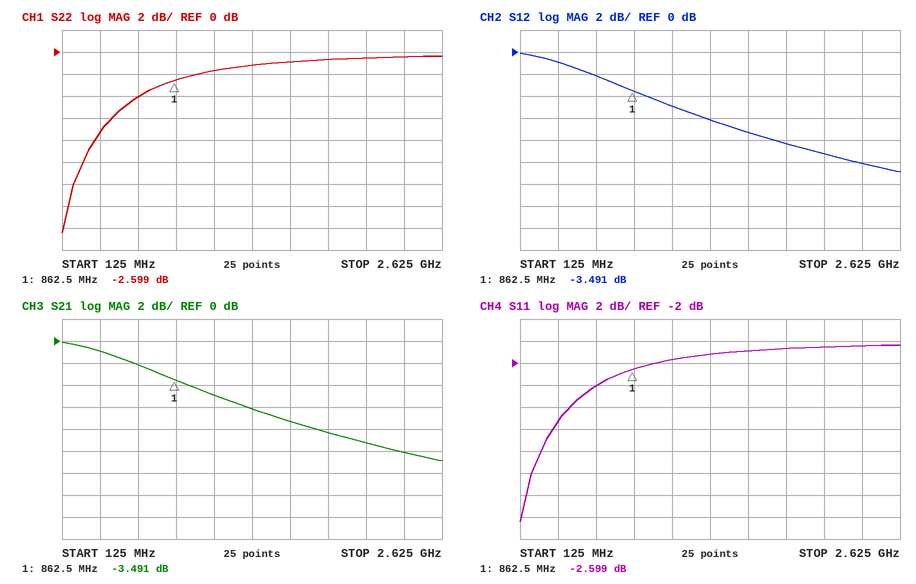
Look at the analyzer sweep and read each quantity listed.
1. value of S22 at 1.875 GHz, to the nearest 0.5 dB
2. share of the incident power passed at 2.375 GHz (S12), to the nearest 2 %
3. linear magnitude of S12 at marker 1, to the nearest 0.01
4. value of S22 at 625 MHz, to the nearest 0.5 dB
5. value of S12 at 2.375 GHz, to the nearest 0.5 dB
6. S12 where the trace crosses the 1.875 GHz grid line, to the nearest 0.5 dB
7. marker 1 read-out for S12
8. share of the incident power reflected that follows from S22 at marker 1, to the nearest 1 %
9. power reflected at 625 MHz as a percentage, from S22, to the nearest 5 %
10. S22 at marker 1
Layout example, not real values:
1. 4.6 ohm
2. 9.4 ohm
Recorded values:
1. -0.5 dB
2. 10 %
3. 0.67
4. -4.0 dB
5. -10.0 dB
6. -8.5 dB
7. -3.491 dB
8. 55 %
9. 40 %
10. -2.599 dB
